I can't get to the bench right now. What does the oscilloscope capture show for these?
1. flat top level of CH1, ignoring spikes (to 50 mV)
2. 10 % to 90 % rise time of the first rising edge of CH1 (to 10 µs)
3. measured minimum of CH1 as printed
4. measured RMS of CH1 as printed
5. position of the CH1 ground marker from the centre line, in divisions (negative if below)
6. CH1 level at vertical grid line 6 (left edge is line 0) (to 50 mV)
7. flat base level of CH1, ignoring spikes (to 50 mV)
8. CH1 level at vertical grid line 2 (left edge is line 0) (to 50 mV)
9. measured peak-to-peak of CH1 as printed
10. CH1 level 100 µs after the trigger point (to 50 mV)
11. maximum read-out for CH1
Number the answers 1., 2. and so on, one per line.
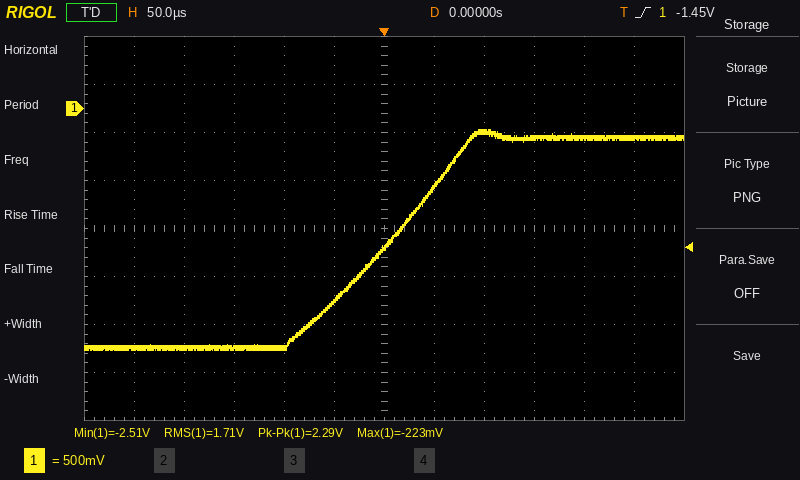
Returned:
1. -300 mV
2. 150 µs
3. -2.51 V
4. 1.71 V
5. +2.5 div
6. -1.45 V
7. -2.50 V
8. -2.50 V
9. 2.29 V
10. -250 mV
11. -223 mV
